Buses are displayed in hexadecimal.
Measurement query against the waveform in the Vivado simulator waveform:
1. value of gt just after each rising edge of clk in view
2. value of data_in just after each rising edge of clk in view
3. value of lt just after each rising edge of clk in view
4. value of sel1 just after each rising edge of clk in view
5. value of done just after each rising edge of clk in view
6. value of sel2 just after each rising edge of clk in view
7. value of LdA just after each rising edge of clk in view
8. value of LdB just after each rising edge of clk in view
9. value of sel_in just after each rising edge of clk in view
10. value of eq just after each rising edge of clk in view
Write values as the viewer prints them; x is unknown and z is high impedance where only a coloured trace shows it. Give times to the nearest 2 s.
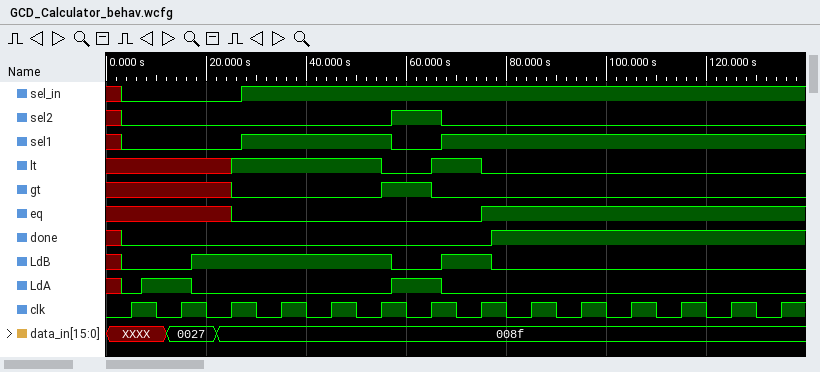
x x 0 0 0 1 0 0 0 0 0 0 0 0
XXXX, 0027, 008f, 008f, 008f, 008f, 008f, 008f, 008f, 008f, 008f, 008f, 008f, 008f
x x 1 1 1 0 1 0 0 0 0 0 0 0
0 0 0 1 1 1 0 1 1 1 1 1 1 1
0 0 0 0 0 0 0 0 1 1 1 1 1 1
0 0 0 0 0 0 1 0 0 0 0 0 0 0
0 1 0 0 0 0 1 0 0 0 0 0 0 0
0 0 1 1 1 1 0 1 0 0 0 0 0 0
0 0 0 1 1 1 1 1 1 1 1 1 1 1
x x 0 0 0 0 0 1 1 1 1 1 1 1
